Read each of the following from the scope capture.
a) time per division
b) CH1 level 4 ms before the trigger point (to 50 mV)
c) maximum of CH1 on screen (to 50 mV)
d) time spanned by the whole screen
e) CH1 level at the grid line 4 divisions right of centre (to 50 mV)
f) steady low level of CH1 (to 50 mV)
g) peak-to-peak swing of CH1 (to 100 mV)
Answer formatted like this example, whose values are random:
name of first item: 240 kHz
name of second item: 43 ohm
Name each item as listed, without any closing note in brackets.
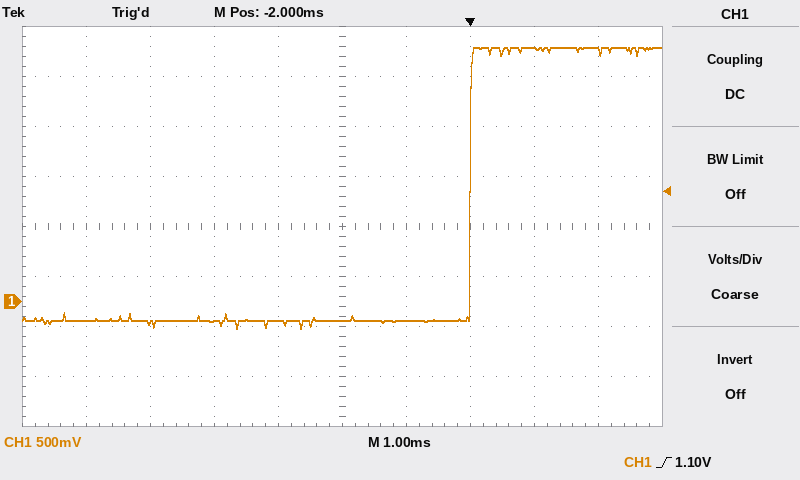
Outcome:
time per division: 1 ms
CH1 level 4 ms before the trigger point: -200 mV
maximum of CH1 on screen: 2.55 V
time spanned by the whole screen: 10 ms
CH1 level at the grid line 4 divisions right of centre: 2.50 V
steady low level of CH1: -200 mV
peak-to-peak swing of CH1: 2.80 V
